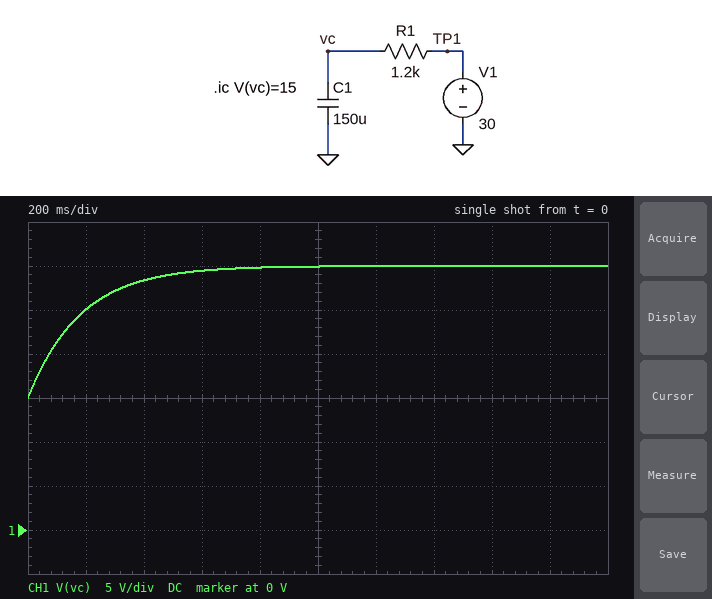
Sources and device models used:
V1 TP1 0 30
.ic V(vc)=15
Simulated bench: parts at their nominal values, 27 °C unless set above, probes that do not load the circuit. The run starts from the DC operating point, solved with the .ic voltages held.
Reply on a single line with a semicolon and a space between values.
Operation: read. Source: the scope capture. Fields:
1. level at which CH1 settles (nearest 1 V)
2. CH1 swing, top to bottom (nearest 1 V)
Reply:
30 V; 15 V
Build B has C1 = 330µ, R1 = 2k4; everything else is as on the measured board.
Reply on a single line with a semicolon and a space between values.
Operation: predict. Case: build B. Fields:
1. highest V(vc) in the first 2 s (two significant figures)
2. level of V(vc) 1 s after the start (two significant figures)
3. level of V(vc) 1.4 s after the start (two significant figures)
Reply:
29 V; 26 V; 27 V
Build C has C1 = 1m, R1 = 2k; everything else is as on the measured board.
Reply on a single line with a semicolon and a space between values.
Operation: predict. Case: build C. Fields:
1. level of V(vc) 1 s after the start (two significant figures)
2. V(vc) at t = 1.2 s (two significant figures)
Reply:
21 V; 22 V
